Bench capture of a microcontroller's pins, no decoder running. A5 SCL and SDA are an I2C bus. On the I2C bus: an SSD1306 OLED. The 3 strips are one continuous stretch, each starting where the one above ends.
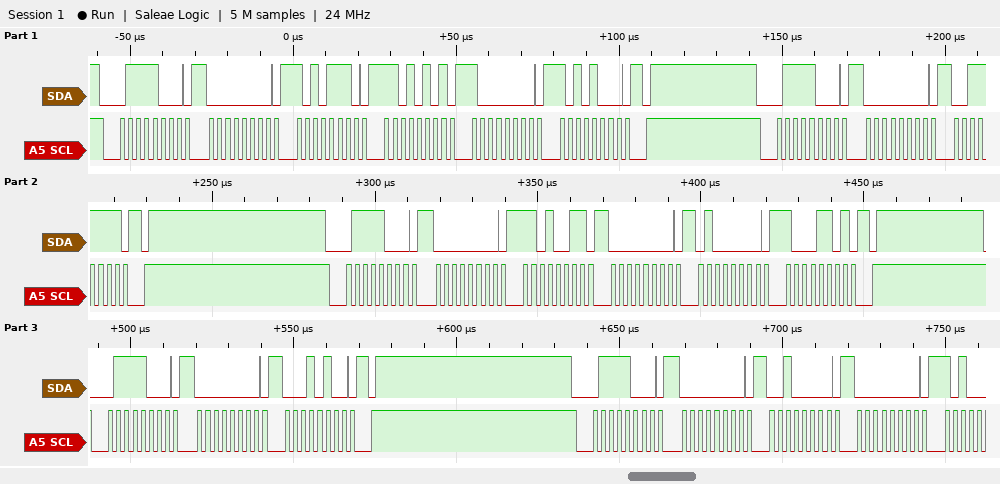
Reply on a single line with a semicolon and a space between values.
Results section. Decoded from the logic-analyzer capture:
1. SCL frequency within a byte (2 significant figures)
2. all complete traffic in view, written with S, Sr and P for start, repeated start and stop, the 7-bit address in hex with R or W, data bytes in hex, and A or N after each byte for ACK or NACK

400 kHz; S 3CW A 00 A AE A D5 A 80 A A8 A P S 3CW A 00 A 3F A P S 3CW A 00 A D3 A 00 A 40 A 8D A P S 3CW A 00 A 14 A P S 3CW A 00 A 20 A 00 A
